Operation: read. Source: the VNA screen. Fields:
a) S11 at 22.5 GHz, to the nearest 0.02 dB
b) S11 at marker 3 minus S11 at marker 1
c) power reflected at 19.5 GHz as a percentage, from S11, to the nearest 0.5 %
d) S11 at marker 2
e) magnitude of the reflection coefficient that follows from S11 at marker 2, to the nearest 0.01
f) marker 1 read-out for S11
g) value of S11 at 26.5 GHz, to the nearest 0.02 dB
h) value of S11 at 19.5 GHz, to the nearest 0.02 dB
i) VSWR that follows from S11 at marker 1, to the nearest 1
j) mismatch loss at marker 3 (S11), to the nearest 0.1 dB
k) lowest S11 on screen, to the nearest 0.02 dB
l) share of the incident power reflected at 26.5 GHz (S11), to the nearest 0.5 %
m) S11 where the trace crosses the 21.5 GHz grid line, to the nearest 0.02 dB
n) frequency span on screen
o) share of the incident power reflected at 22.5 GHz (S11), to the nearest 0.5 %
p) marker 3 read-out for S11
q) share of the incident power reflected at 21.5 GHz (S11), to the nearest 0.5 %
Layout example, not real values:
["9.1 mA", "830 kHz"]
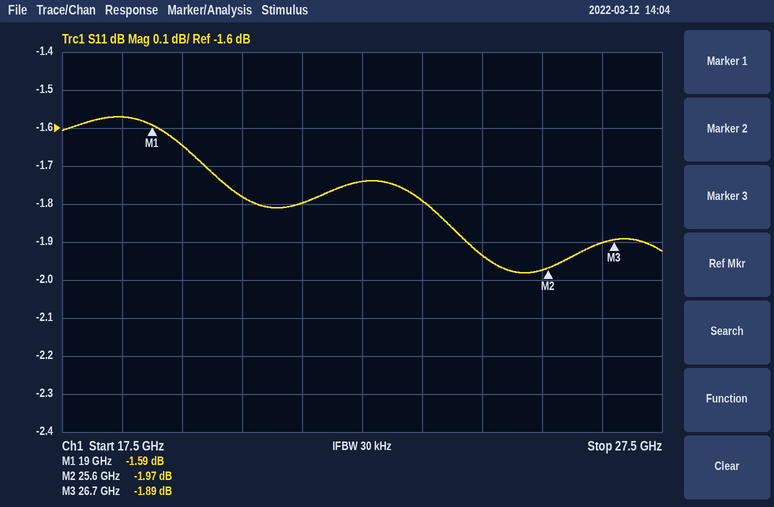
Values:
["-1.74 dB", "-0.30 dB", "68.5 %", "-1.97 dB", "0.80", "-1.59 dB", "-1.90 dB", "-1.64 dB", "11", "4.5 dB", "-1.98 dB", "64.5 %", "-1.80 dB", "10 GHz", "67.0 %", "-1.89 dB", "66.0 %"]
